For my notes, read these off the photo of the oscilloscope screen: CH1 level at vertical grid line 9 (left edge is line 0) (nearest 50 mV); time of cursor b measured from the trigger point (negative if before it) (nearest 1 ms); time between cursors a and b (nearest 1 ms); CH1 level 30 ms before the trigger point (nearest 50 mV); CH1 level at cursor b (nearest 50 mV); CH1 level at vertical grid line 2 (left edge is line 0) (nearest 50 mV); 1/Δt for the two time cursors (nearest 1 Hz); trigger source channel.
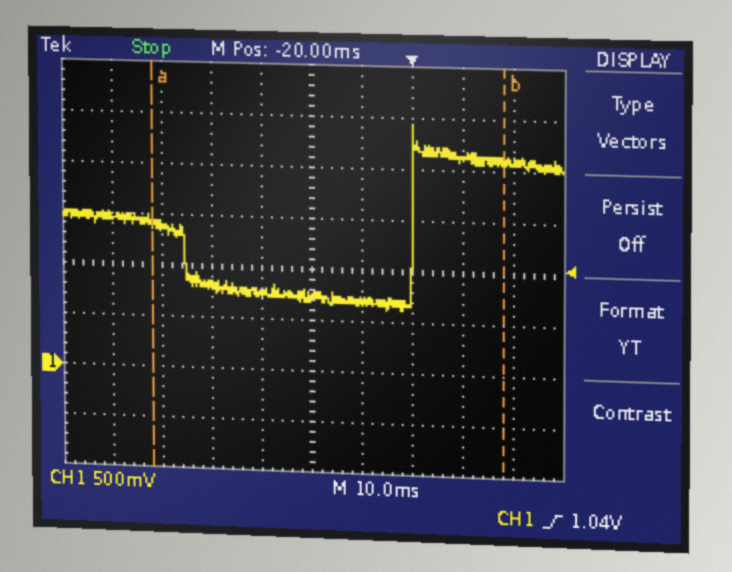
2.10 V
+18 ms
70 ms
750 mV
2.10 V
1.40 V
14 Hz
CH1
